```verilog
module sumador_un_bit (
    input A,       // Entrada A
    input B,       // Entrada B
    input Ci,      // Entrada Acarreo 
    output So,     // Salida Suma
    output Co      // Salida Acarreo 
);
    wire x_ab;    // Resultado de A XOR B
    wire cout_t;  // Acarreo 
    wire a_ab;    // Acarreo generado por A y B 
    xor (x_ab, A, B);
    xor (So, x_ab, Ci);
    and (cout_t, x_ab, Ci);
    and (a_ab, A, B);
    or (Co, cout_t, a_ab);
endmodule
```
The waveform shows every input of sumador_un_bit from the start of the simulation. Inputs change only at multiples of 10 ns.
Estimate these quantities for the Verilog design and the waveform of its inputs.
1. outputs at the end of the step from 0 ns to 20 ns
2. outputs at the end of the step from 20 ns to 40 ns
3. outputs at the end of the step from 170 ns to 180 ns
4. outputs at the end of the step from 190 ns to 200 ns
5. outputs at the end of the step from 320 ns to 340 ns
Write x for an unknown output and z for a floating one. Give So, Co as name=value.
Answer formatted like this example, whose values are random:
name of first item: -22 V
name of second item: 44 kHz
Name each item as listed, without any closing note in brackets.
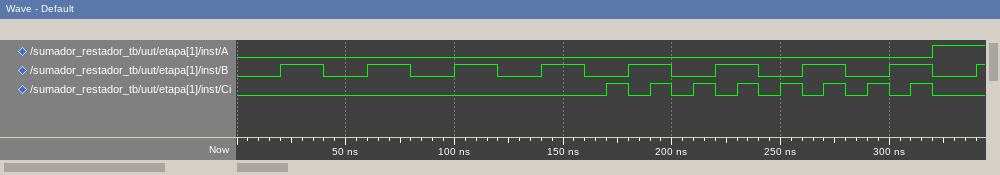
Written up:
outputs at the end of the step from 0 ns to 20 ns: So=0, Co=0
outputs at the end of the step from 20 ns to 40 ns: So=1, Co=0
outputs at the end of the step from 170 ns to 180 ns: So=1, Co=0
outputs at the end of the step from 190 ns to 200 ns: So=0, Co=1
outputs at the end of the step from 320 ns to 340 ns: So=1, Co=0
